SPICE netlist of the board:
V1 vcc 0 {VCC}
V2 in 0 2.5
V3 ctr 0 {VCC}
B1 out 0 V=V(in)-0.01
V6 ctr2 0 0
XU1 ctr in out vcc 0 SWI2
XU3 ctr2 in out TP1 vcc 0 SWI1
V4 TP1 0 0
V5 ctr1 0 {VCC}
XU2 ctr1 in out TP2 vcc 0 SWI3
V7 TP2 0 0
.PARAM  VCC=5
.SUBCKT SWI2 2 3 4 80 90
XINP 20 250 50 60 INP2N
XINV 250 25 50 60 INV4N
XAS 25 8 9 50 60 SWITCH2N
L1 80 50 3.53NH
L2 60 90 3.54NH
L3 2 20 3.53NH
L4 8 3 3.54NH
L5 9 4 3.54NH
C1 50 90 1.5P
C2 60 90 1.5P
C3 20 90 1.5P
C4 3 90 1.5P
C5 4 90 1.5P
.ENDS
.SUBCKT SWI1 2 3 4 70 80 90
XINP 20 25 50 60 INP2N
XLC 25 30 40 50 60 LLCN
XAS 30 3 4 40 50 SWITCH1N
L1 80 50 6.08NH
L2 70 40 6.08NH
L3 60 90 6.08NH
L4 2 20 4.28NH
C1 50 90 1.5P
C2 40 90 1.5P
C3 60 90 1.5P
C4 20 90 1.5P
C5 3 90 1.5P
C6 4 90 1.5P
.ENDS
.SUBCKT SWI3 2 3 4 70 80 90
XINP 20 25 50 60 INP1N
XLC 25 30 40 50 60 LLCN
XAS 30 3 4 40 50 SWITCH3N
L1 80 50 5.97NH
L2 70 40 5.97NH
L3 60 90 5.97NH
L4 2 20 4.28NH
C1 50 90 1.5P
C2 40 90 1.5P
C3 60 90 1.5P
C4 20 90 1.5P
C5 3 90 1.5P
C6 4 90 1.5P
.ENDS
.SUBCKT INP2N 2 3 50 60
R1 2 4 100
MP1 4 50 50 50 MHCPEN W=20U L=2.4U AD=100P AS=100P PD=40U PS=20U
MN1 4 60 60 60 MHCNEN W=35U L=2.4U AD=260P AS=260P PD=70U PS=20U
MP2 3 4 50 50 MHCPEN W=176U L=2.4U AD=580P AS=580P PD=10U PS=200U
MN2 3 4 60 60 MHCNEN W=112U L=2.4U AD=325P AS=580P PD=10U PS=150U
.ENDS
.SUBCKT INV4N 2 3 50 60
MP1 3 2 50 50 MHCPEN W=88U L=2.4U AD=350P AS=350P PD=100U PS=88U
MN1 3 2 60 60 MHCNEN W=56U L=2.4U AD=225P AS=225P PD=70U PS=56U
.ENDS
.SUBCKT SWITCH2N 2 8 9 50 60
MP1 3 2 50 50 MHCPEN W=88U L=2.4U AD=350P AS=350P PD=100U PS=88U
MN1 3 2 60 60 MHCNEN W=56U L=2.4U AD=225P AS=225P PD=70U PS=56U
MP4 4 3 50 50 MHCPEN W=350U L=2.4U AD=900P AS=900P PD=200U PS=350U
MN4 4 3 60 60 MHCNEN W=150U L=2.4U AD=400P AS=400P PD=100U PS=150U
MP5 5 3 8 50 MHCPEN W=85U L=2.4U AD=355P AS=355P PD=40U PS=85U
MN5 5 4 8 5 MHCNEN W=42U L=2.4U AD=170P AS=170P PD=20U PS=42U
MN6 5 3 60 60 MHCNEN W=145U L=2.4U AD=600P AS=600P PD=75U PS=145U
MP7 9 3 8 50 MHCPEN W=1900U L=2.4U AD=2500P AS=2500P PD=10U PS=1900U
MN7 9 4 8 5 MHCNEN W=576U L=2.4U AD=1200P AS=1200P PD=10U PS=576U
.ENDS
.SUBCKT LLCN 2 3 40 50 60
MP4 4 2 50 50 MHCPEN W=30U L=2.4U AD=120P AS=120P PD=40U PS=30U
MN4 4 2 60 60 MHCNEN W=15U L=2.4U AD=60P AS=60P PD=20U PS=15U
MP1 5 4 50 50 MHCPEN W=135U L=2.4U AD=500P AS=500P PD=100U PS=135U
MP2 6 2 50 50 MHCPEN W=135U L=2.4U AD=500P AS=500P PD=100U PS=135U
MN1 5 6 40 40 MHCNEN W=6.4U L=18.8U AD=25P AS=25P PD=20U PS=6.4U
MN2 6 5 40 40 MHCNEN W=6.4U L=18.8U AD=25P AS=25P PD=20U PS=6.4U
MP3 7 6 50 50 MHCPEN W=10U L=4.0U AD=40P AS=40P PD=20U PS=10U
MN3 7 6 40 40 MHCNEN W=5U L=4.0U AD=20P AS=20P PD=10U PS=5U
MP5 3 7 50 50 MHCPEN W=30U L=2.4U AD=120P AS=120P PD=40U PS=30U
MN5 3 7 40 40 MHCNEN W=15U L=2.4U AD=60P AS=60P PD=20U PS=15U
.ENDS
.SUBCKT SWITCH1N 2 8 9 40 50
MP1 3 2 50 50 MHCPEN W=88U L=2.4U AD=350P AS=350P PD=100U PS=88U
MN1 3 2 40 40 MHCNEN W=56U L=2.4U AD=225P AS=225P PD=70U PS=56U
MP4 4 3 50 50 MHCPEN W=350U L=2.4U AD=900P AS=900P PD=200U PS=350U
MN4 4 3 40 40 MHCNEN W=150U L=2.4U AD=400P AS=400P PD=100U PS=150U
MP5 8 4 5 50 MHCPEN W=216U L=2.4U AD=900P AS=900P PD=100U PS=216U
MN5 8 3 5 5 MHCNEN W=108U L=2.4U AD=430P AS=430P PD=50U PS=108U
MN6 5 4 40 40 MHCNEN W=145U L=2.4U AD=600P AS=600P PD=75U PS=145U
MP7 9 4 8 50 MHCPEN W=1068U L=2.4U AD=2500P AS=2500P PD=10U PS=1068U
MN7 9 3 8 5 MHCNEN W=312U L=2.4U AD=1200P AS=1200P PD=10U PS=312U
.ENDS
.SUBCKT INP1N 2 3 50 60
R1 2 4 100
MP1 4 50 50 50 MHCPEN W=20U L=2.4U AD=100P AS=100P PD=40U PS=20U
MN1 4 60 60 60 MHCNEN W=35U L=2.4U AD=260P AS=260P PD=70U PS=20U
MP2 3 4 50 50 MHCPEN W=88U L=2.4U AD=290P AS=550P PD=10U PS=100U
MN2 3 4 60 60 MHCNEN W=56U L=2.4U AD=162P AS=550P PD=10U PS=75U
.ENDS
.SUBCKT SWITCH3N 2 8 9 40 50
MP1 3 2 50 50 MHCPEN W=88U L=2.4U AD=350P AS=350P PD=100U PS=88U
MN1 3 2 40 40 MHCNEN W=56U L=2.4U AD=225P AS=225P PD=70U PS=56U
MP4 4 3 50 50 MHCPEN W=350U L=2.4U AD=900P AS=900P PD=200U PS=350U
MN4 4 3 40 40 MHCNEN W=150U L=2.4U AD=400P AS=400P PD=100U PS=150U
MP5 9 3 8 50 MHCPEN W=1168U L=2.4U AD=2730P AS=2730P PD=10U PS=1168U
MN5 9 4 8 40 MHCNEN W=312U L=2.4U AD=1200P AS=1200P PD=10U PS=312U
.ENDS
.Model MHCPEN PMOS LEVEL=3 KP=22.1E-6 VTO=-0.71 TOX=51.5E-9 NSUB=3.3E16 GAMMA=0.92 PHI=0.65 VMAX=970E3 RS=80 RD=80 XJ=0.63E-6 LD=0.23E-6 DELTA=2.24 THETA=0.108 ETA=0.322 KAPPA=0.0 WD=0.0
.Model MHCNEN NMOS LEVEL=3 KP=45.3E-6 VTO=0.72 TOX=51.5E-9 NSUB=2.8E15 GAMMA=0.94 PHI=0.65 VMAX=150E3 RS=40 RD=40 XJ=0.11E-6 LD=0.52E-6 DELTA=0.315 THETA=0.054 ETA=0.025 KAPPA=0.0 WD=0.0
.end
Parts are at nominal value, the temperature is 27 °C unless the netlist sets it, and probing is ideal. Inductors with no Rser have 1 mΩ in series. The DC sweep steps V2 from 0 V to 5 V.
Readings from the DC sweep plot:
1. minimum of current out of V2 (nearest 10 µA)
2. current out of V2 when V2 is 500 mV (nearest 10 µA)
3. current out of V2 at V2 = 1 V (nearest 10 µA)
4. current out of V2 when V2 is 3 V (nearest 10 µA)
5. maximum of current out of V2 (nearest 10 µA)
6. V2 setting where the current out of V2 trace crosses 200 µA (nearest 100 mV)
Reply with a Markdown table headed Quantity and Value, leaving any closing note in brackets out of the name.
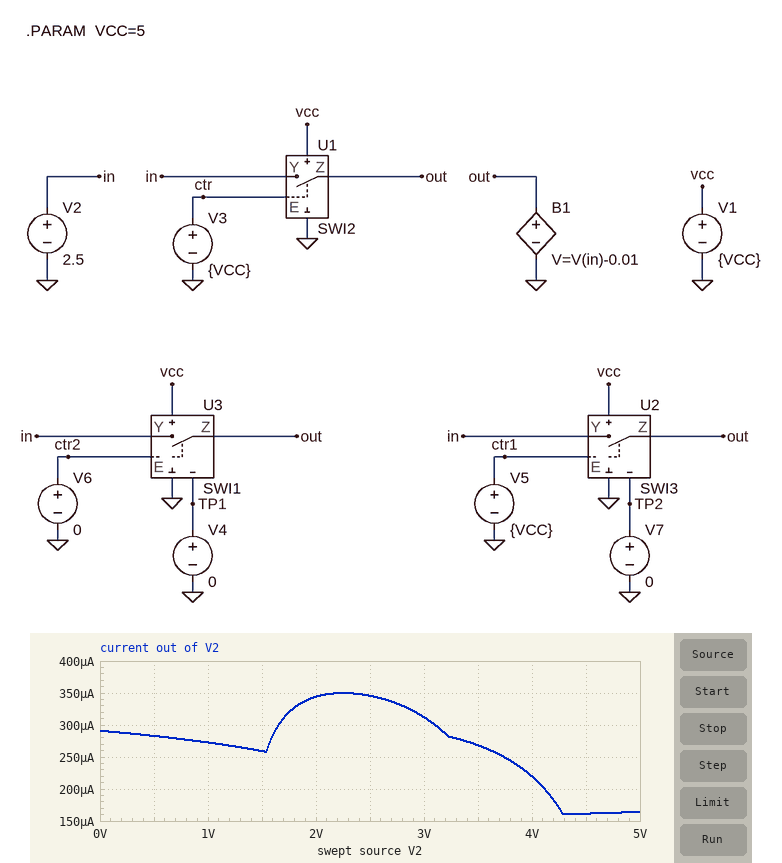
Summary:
| Quantity | Value |
|---|---|
| minimum of current out of V2 | 160 µA |
| current out of V2 when V2 is 500 mV | 280 µA |
| current out of V2 at V2 = 1 V | 270 µA |
| current out of V2 when V2 is 3 V | 310 µA |
| maximum of current out of V2 | 350 µA |
| V2 setting where the current out of V2 trace crosses 200 µA | 4.1 V |
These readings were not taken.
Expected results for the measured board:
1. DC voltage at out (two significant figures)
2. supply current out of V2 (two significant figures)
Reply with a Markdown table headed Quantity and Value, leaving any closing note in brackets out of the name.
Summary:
| Quantity | Value |
|---|---|
| DC voltage at out | 2.5 V |
| supply current out of V2 | 350 µA |
